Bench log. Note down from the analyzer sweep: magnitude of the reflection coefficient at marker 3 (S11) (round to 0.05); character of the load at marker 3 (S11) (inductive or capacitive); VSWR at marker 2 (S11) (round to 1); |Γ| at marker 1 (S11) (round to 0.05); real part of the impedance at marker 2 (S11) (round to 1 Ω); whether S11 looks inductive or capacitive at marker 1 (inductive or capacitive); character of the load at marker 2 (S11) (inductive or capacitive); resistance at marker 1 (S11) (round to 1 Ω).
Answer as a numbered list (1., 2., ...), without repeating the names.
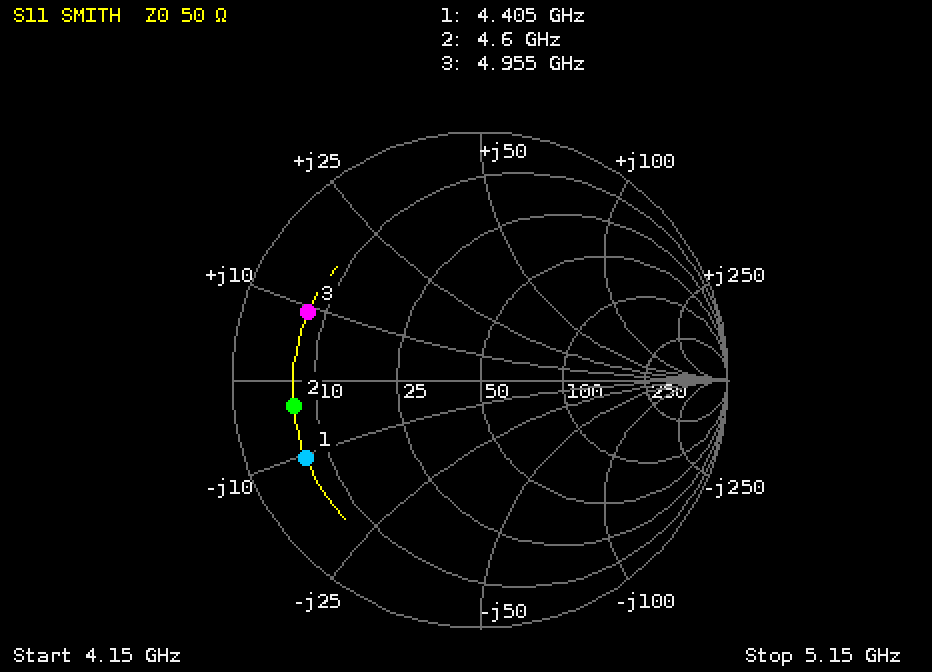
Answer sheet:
1. 0.75
2. inductive
3. 7
4. 0.75
5. 7 Ω
6. capacitive
7. capacitive
8. 7 Ω
